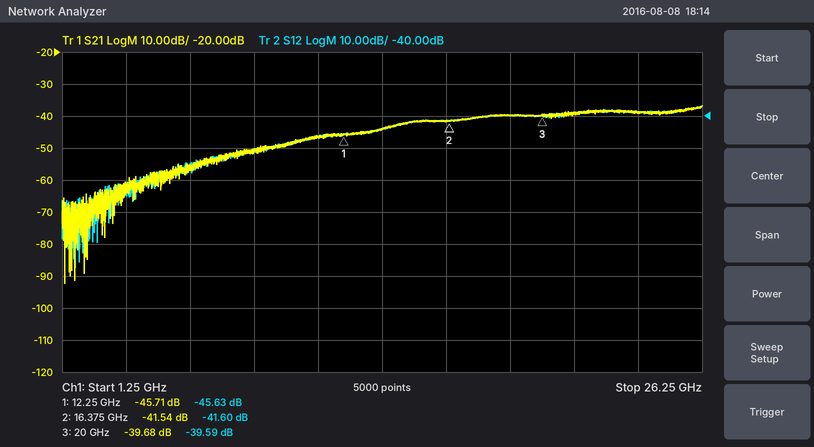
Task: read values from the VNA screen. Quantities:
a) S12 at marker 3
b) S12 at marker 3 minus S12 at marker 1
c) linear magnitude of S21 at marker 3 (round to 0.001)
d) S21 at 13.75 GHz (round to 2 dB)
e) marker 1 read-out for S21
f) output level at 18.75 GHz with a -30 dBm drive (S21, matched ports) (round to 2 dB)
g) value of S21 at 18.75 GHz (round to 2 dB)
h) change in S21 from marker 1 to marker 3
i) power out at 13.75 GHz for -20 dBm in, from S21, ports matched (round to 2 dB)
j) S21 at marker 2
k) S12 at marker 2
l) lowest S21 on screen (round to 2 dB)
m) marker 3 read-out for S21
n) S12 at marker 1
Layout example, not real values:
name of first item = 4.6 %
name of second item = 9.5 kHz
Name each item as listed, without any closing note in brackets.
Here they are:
S12 at marker 3 = -39.59 dB
S12 at marker 3 minus S12 at marker 1 = 6.04 dB
linear magnitude of S21 at marker 3 = 0.010
S21 at 13.75 GHz = -44 dB
marker 1 read-out for S21 = -45.71 dB
output level at 18.75 GHz with a -30 dBm drive (S21, matched ports) = -70 dBm
value of S21 at 18.75 GHz = -40 dB
change in S21 from marker 1 to marker 3 = 6.03 dB
power out at 13.75 GHz for -20 dBm in, from S21, ports matched = -64 dBm
S21 at marker 2 = -41.54 dB
S12 at marker 2 = -41.60 dB
lowest S21 on screen = -92 dB
marker 3 read-out for S21 = -39.68 dB
S12 at marker 1 = -45.63 dB
